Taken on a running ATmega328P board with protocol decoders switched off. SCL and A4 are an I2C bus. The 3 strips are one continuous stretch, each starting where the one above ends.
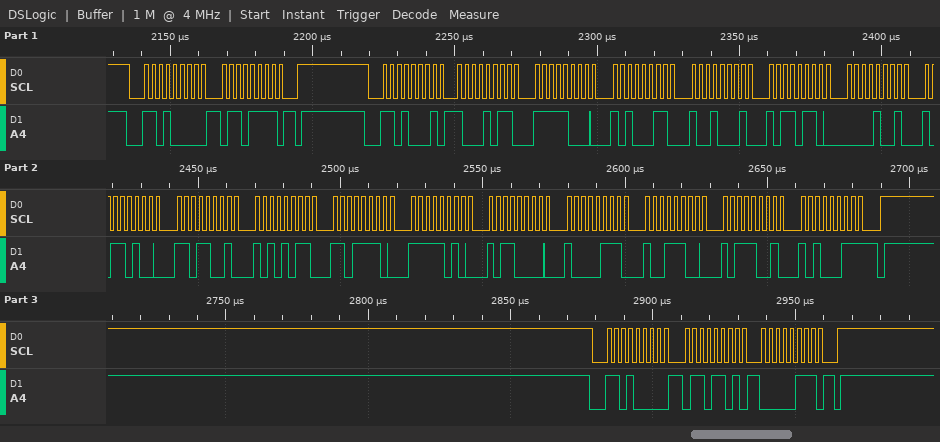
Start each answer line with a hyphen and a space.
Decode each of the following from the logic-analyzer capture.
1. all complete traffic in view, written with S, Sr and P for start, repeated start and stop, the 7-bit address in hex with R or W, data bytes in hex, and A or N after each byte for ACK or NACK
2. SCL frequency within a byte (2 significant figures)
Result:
- S 68W A 6F A P S 68R A 8B A F8 A A3 A 91 A B6 A 09 A B4 A D9 A AB A DE A FA A B0 A 87 A 9C A B9 A A3 N P S 68W A 6D A 07 A P
- 400 kHz
